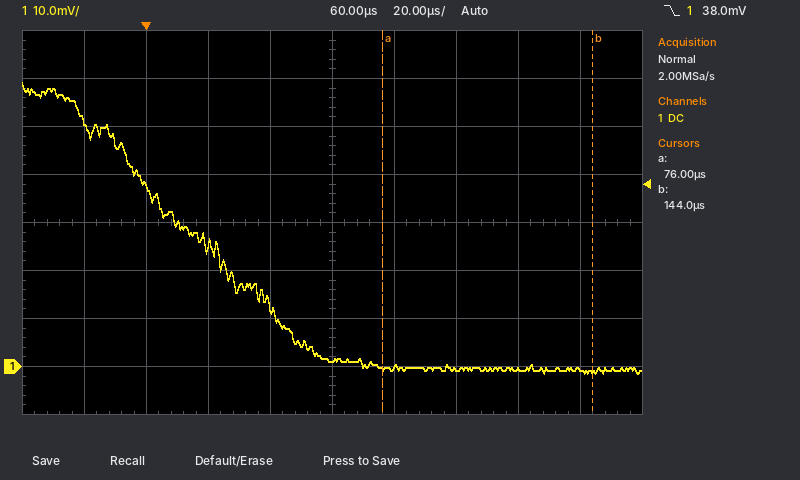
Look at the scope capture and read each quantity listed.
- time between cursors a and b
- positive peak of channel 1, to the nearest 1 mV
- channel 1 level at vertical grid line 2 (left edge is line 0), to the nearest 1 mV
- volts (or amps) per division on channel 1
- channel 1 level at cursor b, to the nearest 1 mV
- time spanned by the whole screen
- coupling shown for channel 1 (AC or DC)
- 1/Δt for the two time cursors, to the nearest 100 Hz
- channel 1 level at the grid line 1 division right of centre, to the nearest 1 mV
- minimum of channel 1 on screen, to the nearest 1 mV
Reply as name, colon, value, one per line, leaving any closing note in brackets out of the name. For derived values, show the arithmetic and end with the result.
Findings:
time between cursors a and b: 144 µs − (76 µs) = 68 µs
positive peak of channel 1, to the nearest 1 mV: 59 mV
channel 1 level at vertical grid line 2 (left edge is line 0), to the nearest 1 mV: 38 mV
volts (or amps) per division on channel 1: 10 mV
channel 1 level at cursor b, to the nearest 1 mV: -1 mV
time spanned by the whole screen: 200 µs
coupling shown for channel 1: DC
1/Δt for the two time cursors, to the nearest 100 Hz: 1 / 68 µs ≈ 14.7 kHz
channel 1 level at the grid line 1 division right of centre, to the nearest 1 mV: 0 mV
minimum of channel 1 on screen, to the nearest 1 mV: -1 mV
